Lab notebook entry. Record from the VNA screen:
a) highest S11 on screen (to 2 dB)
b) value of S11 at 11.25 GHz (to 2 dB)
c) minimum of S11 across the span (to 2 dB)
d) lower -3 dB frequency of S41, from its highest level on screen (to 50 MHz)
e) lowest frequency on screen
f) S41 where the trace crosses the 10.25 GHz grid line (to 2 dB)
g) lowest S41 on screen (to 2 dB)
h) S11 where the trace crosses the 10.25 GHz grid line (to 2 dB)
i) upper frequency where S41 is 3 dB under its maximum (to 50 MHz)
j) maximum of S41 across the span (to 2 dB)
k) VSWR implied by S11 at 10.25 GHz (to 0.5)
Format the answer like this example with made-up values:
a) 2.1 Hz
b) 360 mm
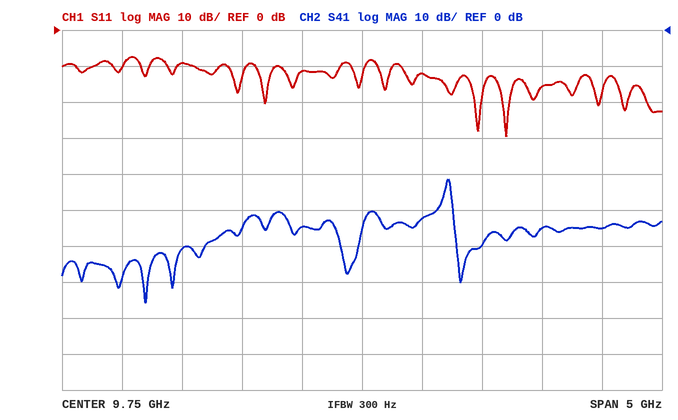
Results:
a) -8 dB
b) -16 dB
c) -30 dB
d) 10.45 GHz
e) 7.25 GHz
f) -52 dB
g) -76 dB
h) -12 dB
i) 10.50 GHz
j) -42 dB
k) 1.5
